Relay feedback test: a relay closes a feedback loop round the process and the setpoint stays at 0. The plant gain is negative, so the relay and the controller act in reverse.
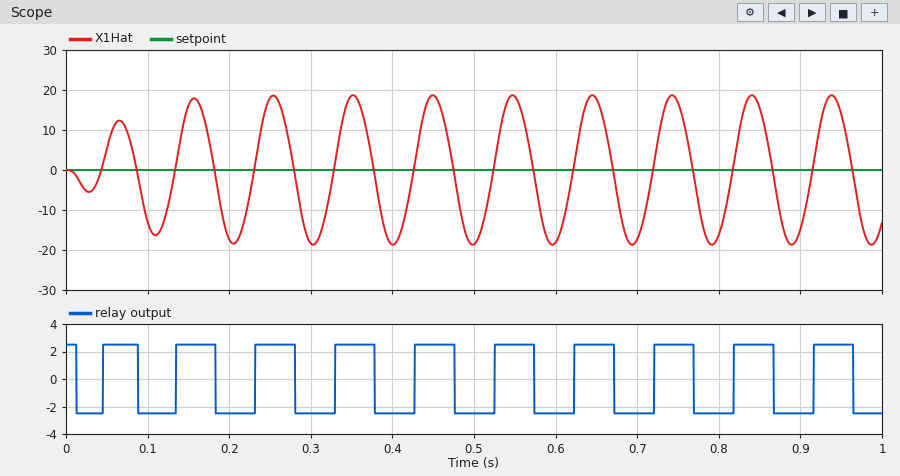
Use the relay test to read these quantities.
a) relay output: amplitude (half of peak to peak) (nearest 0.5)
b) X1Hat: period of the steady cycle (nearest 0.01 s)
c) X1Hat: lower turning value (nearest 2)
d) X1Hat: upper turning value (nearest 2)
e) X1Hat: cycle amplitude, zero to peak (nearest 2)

2.5
0.10 s
-18
18
18
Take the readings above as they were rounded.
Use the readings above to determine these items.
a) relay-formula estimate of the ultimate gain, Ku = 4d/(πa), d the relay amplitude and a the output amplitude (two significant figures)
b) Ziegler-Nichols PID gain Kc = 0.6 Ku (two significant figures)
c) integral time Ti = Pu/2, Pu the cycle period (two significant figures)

0.18
0.11
0.050 s
